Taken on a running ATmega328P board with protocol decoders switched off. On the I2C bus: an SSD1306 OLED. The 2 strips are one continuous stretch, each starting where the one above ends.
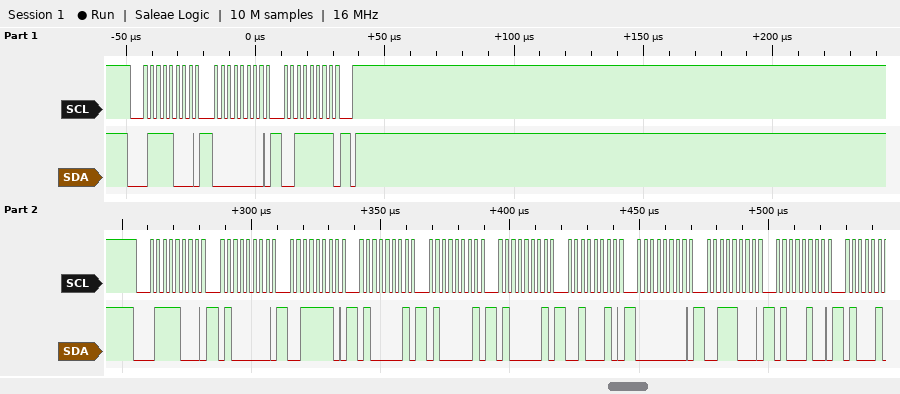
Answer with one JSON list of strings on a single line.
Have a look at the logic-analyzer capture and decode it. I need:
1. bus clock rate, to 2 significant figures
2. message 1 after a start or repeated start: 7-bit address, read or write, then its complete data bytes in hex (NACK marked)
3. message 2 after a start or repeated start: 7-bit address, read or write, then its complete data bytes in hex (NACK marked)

["400 kHz", "0x3C write: 00 3F", "0x3C write: 40 3E 41 41 41 22 00 38 44"]
